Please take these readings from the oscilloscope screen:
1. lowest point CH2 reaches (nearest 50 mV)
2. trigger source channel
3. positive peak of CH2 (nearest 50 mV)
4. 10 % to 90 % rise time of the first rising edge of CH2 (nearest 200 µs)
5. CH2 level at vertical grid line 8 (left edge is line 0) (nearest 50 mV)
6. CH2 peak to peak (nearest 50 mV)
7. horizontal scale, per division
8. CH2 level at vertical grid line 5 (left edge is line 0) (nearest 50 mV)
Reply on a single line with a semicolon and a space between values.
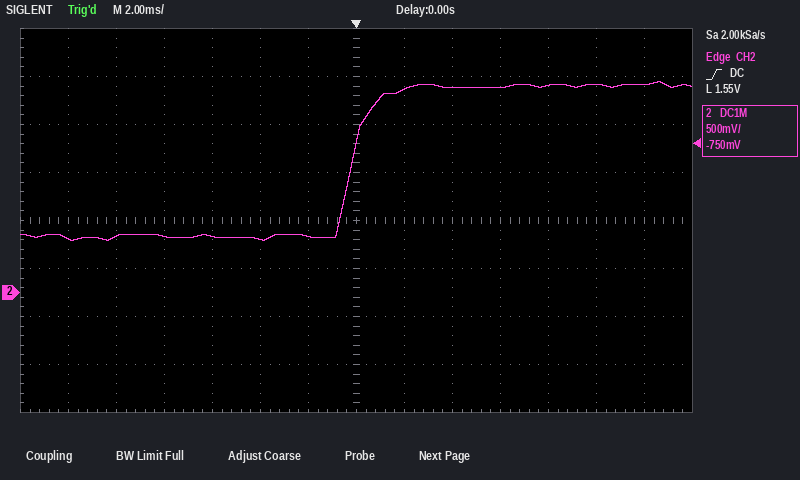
550 mV; CH2; 2.20 V; 1.6 ms; 2.10 V; 1.65 V; 2 ms; 550 mV
